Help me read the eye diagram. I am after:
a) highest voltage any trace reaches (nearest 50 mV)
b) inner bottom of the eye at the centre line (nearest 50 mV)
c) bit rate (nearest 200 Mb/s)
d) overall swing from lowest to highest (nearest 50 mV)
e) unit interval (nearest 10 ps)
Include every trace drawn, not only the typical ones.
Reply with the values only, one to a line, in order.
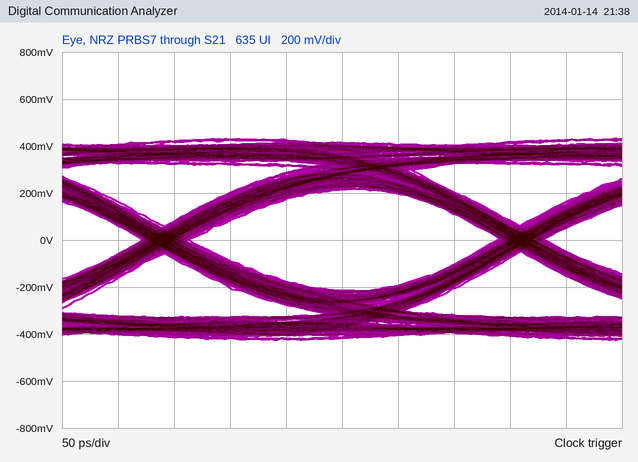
450 mV
-200 mV
3.2 Gb/s
850 mV
320 ps
